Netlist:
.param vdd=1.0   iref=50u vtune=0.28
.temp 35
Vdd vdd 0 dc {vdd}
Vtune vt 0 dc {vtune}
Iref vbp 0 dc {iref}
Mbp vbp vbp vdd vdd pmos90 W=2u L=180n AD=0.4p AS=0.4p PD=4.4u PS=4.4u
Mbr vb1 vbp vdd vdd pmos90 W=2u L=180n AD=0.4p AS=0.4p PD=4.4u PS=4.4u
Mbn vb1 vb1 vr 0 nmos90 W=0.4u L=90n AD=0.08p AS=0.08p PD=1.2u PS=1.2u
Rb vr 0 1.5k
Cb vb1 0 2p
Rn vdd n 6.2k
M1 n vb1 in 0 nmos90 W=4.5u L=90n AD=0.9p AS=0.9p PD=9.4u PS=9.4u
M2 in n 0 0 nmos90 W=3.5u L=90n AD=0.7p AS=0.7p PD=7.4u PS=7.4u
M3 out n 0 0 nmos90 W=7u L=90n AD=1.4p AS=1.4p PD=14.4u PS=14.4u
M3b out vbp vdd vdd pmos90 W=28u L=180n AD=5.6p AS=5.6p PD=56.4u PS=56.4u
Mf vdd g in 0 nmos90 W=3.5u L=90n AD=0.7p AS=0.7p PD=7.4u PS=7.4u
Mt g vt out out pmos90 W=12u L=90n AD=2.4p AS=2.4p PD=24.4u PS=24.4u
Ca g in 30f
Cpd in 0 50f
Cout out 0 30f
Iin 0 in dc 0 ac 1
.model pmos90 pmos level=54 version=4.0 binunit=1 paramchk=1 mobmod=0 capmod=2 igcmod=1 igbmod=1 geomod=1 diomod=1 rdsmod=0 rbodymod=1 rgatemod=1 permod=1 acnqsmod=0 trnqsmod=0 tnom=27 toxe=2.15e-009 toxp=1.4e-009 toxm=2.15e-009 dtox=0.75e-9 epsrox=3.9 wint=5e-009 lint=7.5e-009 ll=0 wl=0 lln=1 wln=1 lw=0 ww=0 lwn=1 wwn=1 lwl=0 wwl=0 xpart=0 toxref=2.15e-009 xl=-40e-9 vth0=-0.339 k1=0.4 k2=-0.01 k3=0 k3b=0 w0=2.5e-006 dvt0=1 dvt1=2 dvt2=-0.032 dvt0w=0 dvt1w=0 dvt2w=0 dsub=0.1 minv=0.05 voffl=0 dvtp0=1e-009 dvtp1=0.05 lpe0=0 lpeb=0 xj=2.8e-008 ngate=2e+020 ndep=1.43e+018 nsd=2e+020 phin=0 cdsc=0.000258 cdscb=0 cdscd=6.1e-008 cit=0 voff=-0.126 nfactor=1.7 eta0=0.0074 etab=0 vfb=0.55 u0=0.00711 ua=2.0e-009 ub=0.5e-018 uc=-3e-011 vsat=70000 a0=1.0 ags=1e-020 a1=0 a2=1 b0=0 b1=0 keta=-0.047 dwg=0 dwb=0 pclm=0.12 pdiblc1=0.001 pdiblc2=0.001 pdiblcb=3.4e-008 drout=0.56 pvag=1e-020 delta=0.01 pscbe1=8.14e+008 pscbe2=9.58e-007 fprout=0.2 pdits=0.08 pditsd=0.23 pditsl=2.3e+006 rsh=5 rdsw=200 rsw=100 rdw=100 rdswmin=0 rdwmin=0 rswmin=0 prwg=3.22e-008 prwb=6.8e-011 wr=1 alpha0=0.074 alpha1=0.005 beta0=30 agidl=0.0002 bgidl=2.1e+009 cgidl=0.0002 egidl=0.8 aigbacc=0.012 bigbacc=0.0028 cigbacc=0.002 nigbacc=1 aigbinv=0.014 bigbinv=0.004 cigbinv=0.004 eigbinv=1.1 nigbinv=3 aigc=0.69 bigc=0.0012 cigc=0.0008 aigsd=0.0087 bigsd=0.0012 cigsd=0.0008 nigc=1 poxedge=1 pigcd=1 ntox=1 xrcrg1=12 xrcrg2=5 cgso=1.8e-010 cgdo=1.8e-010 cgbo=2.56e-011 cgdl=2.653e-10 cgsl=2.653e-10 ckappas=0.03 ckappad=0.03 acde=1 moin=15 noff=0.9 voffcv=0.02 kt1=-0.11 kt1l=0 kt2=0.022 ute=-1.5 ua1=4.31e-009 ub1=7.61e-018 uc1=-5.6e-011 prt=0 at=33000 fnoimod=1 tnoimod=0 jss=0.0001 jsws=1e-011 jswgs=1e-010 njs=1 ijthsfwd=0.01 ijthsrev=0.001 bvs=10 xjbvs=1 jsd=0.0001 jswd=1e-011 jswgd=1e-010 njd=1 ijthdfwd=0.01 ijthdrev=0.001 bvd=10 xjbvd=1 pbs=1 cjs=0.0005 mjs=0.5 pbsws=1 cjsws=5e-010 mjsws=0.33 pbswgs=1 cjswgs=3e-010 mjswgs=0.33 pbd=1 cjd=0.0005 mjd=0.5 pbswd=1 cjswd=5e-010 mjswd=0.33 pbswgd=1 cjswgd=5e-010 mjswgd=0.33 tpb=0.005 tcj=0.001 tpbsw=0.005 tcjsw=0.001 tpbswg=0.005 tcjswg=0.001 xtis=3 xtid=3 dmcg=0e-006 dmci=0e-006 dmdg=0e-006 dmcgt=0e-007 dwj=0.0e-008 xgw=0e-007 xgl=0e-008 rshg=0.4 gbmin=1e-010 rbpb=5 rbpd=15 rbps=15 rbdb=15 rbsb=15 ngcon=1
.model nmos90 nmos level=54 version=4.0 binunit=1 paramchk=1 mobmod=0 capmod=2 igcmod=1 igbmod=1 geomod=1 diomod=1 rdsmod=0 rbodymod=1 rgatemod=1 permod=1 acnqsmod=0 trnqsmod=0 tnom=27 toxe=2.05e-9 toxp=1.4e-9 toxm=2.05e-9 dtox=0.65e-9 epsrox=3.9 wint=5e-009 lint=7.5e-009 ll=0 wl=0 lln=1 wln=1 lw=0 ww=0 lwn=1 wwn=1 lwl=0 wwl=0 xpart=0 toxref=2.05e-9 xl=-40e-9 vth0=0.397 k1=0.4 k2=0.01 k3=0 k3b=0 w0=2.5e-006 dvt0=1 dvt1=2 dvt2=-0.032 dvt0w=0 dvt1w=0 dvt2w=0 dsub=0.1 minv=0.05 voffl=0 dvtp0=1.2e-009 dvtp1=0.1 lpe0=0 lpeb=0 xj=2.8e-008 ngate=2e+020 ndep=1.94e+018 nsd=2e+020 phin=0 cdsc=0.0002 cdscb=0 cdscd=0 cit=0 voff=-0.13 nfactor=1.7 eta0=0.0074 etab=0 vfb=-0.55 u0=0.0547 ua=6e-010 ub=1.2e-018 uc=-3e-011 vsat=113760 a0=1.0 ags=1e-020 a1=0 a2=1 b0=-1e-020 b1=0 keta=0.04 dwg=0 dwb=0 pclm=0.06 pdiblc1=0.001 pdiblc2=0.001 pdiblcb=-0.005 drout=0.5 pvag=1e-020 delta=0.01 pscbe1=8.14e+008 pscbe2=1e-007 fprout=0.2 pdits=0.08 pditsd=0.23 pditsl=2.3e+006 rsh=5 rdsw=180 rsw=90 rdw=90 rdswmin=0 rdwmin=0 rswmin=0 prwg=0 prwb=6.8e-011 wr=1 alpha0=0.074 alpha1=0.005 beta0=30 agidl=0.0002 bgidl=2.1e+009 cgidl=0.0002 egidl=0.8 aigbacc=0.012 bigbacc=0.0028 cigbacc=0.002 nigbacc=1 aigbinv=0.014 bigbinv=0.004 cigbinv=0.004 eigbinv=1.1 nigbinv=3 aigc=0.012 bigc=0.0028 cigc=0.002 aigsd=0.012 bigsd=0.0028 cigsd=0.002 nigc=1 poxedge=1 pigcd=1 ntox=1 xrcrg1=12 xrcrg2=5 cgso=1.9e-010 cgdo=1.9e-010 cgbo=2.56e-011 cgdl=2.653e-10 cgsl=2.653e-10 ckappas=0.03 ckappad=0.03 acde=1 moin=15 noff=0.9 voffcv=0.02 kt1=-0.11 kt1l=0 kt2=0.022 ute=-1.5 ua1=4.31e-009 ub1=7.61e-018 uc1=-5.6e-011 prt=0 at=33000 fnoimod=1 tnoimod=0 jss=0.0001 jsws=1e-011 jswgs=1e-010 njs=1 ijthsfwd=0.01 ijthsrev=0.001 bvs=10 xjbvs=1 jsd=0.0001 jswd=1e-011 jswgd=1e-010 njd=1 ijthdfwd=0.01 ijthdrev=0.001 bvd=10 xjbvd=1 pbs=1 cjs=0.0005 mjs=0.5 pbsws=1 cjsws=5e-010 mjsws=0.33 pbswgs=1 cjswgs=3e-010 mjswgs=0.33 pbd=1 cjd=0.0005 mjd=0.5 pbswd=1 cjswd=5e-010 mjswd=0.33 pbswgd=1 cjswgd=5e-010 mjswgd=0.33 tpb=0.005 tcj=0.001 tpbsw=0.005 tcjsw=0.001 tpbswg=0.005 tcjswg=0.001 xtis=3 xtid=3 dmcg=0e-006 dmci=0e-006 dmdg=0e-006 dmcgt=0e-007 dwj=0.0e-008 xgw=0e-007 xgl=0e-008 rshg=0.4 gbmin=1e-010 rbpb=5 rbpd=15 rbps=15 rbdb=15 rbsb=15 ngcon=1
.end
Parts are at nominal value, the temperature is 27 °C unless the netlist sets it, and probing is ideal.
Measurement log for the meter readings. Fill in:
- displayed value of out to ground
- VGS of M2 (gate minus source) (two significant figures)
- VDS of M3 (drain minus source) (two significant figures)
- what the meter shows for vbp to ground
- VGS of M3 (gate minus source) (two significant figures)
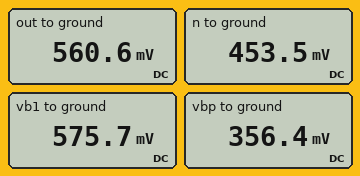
560.6 mV
450 mV
560 mV
356.4 mV
450 mV
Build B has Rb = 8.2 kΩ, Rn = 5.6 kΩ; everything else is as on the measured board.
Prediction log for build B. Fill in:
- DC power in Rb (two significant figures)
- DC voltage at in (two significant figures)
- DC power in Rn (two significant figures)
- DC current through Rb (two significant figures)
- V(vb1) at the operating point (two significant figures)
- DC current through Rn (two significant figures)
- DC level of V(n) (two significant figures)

11 µW
350 mV
60 µW
37 µA
820 mV
100 µA
420 mV
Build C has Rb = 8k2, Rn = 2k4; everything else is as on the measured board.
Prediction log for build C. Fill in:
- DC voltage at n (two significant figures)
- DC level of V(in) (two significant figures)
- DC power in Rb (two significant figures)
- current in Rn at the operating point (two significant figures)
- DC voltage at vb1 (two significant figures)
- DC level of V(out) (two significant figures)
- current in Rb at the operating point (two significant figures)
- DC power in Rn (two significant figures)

450 mV
310 mV
11 µW
230 µA
820 mV
610 mV
37 µA
130 µW
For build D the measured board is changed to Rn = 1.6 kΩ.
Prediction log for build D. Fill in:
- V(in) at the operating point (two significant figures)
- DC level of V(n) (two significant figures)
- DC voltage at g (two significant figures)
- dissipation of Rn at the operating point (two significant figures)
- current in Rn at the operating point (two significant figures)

110 mV
500 mV
200 mV
150 µW
310 µA
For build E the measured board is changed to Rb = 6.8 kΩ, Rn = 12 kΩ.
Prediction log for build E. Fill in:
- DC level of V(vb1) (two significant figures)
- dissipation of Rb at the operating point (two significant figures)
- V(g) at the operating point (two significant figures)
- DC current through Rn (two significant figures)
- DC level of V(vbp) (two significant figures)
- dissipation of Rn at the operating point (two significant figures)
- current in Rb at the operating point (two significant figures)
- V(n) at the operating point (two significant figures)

800 mV
11 µW
790 mV
49 µA
360 mV
29 µW
40 µA
410 mV
